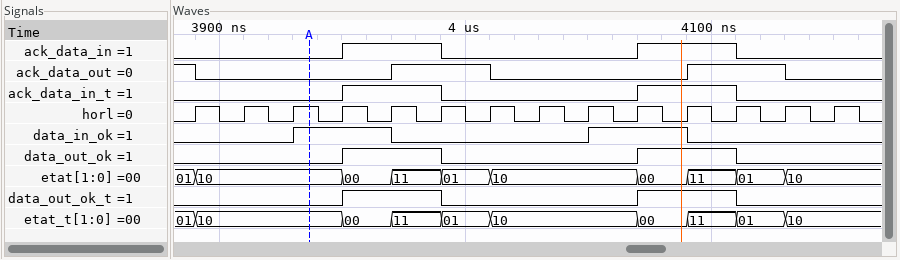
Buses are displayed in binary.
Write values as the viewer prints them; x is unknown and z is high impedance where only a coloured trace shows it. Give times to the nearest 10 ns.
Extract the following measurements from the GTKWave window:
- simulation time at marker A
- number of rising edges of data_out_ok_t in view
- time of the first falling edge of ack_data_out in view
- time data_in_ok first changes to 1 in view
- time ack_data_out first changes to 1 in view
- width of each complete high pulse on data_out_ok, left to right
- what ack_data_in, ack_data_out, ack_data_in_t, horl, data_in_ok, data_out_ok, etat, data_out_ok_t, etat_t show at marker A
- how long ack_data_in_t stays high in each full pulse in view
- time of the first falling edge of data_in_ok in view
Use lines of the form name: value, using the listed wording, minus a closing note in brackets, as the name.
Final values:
simulation time at marker A: 3940 ns
number of rising edges of data_out_ok_t in view: 2
time of the first falling edge of ack_data_out in view: 3890 ns
time data_in_ok first changes to 1 in view: 3930 ns
time ack_data_out first changes to 1 in view: 3970 ns
width of each complete high pulse on data_out_ok, left to right: 40 ns, 40 ns
what ack_data_in, ack_data_out, ack_data_in_t, horl, data_in_ok, data_out_ok, etat, data_out_ok_t, etat_t show at marker A: ack_data_in=0, ack_data_out=0, ack_data_in_t=0, horl=1, data_in_ok=1, data_out_ok=0, etat=10, data_out_ok_t=0, etat_t=10
how long ack_data_in_t stays high in each full pulse in view: 40 ns, 40 ns
time of the first falling edge of data_in_ok in view: 3970 ns
